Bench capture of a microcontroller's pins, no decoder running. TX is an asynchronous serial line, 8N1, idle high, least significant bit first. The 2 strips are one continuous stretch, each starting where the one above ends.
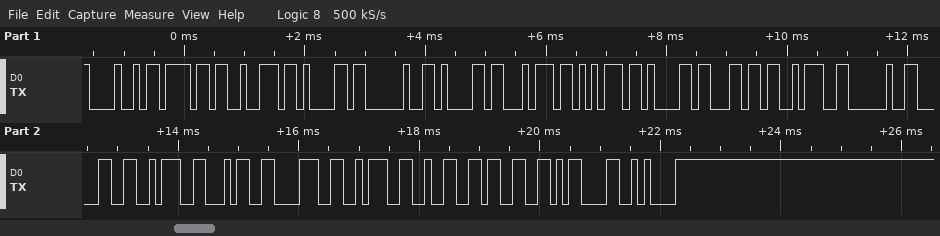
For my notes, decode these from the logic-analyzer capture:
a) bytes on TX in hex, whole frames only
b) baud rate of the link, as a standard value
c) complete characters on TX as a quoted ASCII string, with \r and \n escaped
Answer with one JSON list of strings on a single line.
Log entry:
["48 6F 72 61 20 61 74 75 61 6C 3A 20 30 3A 34 38 3A 32 33 0D 0A", "9600 baud", "\"Hora atual: 0:48:23\\r\\n\""]
